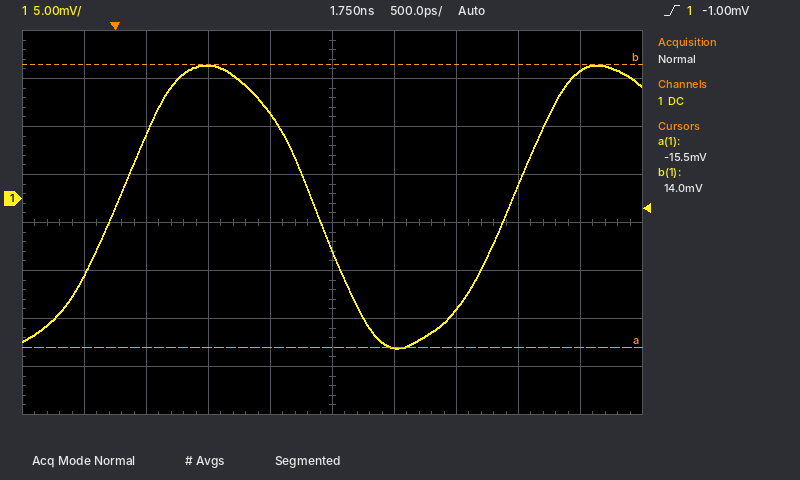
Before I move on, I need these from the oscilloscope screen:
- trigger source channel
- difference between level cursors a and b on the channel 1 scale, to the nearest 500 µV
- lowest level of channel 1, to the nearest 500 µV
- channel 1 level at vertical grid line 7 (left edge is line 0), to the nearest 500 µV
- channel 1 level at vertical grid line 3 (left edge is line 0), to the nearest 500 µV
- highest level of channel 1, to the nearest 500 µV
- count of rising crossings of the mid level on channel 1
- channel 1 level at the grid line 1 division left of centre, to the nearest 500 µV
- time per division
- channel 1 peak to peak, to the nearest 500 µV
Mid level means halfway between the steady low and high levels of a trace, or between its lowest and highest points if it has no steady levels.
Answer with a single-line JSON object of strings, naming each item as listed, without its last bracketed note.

{"trigger source channel": "channel 1", "difference between level cursors a and b on the channel 1 scale, to the nearest 500 µV": "29.5 mV", "lowest level of channel 1, to the nearest 500 µV": "-15.5 mV", "channel 1 level at vertical grid line 7 (left edge is line 0), to the nearest 500 µV": "-11.5 mV", "channel 1 level at vertical grid line 3 (left edge is line 0), to the nearest 500 µV": "14.0 mV", "highest level of channel 1, to the nearest 500 µV": "14.0 mV", "count of rising crossings of the mid level on channel 1": "2", "channel 1 level at the grid line 1 division left of centre, to the nearest 500 µV": "9.0 mV", "time per division": "500 ps", "channel 1 peak to peak, to the nearest 500 µV": "29.5 mV"}
